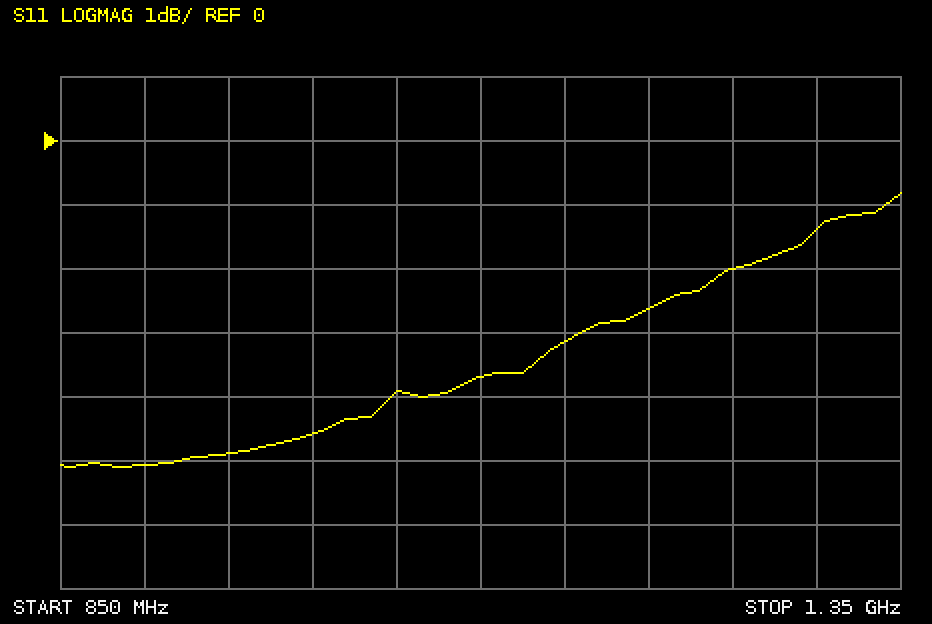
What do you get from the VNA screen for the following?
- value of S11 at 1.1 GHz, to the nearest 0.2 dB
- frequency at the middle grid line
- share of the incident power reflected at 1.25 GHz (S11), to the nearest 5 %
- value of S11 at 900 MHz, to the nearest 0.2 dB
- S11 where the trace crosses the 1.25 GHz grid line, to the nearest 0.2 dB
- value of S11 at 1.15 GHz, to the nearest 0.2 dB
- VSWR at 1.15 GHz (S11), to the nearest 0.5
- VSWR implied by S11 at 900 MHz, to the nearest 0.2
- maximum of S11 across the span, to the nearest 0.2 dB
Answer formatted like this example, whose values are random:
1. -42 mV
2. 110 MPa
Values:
1. -3.6 dB
2. 1.1 GHz
3. 65 %
4. -5.0 dB
5. -2.0 dB
6. -3.2 dB
7. 5.5
8. 3.6
9. -0.8 dB
